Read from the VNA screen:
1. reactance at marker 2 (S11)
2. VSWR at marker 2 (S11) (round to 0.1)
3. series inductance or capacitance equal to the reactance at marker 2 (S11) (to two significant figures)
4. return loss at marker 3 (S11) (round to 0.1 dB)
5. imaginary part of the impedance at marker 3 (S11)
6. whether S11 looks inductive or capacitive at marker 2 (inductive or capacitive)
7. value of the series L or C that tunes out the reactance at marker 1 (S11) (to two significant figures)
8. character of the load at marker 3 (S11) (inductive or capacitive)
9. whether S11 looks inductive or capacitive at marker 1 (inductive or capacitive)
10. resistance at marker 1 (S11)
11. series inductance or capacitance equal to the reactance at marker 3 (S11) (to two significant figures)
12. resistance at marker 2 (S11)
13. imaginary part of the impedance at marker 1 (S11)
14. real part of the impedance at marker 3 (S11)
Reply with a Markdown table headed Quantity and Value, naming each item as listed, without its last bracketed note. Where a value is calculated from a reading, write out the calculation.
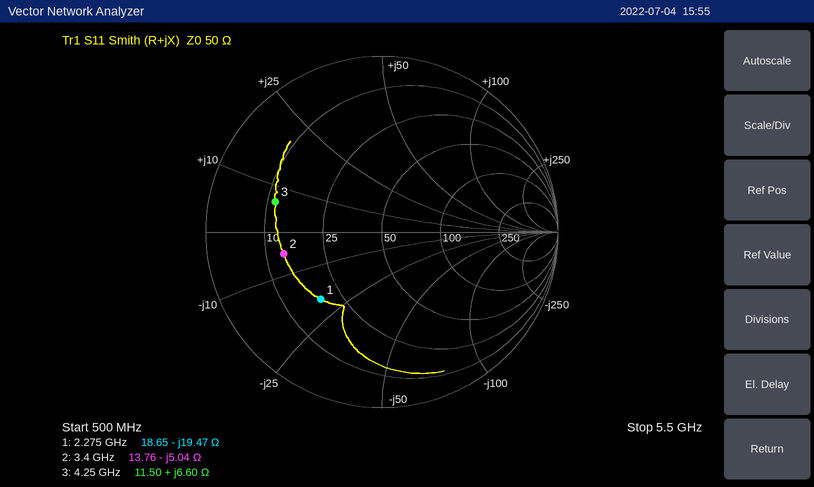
| Quantity | Value |
|---|---|
| reactance at marker 2 | -5.04 Ω |
| VSWR at marker 2 (S11) | 3.7 |
| series inductance or capacitance equal to the reactance at marker 2 (S11) | C = 1/(2π × 3.4 GHz × 5.04 Ω) ≈ 9.3 pF |
| return loss at marker 3 (S11) | 4.0 dB |
| imaginary part of the impedance at marker 3 | +6.60 Ω |
| whether S11 looks inductive or capacitive at marker 2 | capacitive |
| value of the series L or C that tunes out the reactance at marker 1 (S11) | L = 19.47 Ω/(2π × 2.275 GHz) ≈ 1.4 nH |
| character of the load at marker 3 (S11) | inductive |
| whether S11 looks inductive or capacitive at marker 1 | capacitive |
| resistance at marker 1 | 18.65 Ω |
| series inductance or capacitance equal to the reactance at marker 3 (S11) | L = 6.6 Ω/(2π × 4.25 GHz) ≈ 247 pH, so 250 pH to two significant figures |
| resistance at marker 2 | 13.76 Ω |
| imaginary part of the impedance at marker 1 | -19.47 Ω |
| real part of the impedance at marker 3 | 11.50 Ω |
